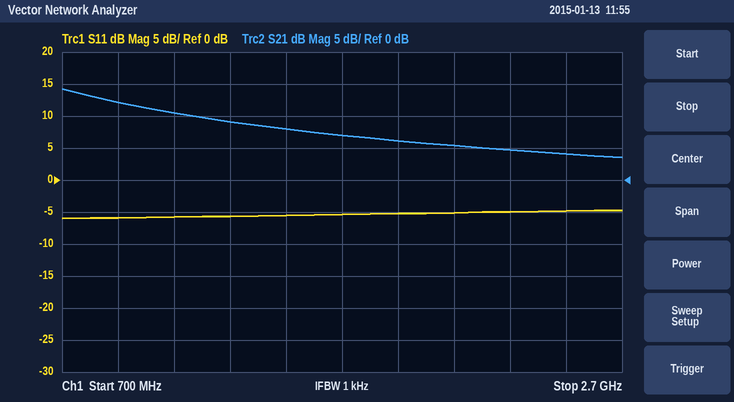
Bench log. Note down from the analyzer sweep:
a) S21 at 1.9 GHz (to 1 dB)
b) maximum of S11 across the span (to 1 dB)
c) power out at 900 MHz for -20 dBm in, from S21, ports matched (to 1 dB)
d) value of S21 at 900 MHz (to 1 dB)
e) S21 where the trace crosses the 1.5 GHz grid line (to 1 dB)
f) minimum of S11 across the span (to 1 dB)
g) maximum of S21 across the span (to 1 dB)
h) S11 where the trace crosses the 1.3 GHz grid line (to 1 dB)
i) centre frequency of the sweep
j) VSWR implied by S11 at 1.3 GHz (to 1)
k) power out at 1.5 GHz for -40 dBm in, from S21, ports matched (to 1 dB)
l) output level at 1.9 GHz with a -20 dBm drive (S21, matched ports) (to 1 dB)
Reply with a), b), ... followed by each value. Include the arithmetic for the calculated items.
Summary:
a) 6 dB
b) -5 dB
c) -20 dBm + (12 dB) = -8 dBm
d) 12 dB
e) 8 dB
f) -6 dB
g) 14 dB
h) -6 dB
i) 1.7 GHz
j) |Γ| = 10^(-6/20) = 0.5012; VSWR = (1 + 0.5012)/(1 − 0.5012) ≈ 3
k) -40 dBm + (8 dB) = -32 dBm
l) -20 dBm + (6 dB) = -14 dBm
